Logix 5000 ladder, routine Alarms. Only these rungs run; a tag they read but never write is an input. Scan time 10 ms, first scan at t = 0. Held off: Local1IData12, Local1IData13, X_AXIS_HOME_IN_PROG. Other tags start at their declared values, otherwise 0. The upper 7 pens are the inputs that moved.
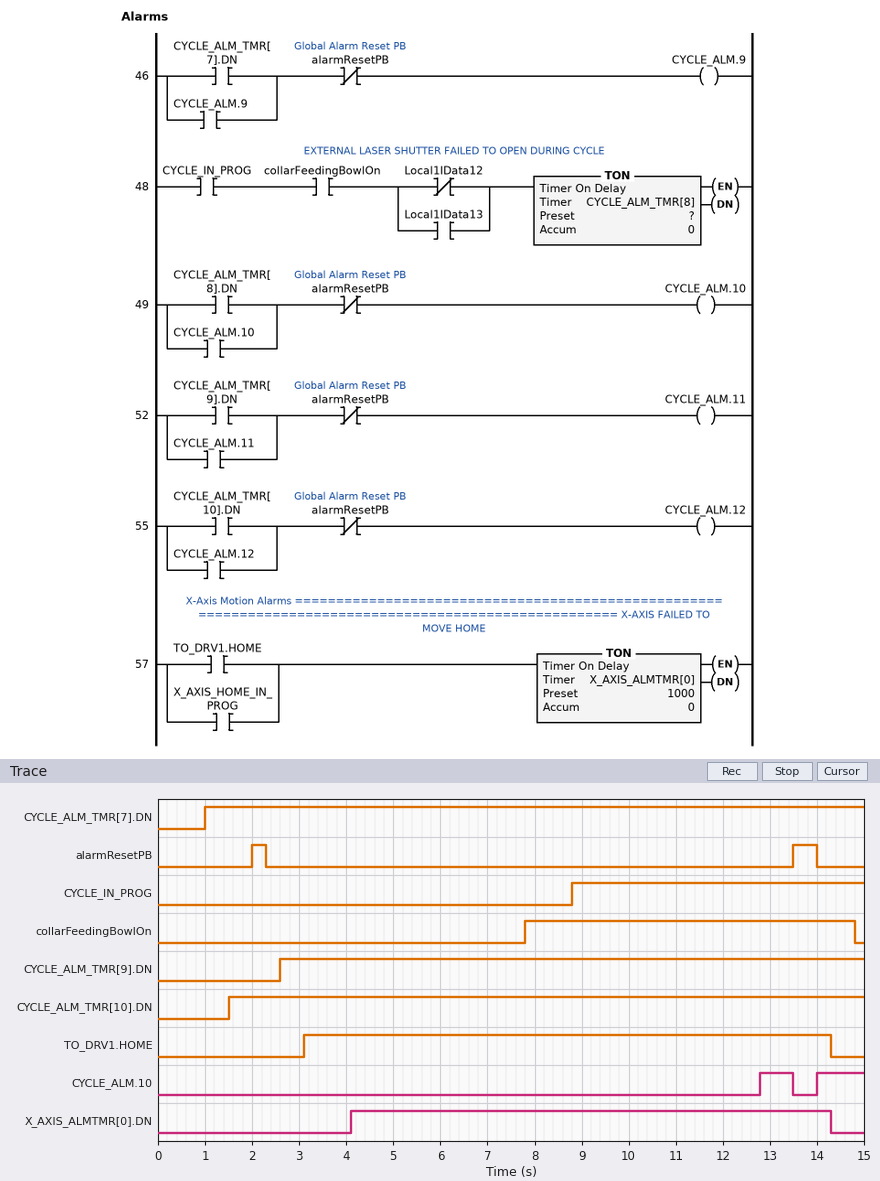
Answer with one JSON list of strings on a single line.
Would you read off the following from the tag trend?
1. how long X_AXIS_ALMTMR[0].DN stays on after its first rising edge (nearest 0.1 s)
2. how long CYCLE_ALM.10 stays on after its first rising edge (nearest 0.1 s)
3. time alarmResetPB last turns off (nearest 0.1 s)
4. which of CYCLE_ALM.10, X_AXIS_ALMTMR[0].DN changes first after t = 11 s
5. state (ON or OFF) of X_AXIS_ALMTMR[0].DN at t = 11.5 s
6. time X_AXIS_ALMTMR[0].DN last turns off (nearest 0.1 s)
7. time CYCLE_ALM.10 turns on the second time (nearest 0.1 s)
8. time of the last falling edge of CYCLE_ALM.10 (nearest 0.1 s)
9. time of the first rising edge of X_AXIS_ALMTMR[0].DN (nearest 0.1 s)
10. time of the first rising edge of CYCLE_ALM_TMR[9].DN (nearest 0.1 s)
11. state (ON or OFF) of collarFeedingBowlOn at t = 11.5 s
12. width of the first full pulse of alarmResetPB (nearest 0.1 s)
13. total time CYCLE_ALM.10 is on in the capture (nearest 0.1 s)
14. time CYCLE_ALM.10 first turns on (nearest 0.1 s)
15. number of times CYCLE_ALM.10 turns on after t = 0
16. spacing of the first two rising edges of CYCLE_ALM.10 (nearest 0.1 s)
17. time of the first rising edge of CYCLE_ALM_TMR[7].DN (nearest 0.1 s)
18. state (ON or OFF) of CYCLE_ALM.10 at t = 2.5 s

["10.2 s", "0.7 s", "14.0 s", "CYCLE_ALM.10", "ON", "14.3 s", "14.0 s", "13.5 s", "4.1 s", "2.6 s", "ON", "0.3 s", "1.7 s", "12.8 s", "2", "1.2 s", "1.0 s", "OFF"]
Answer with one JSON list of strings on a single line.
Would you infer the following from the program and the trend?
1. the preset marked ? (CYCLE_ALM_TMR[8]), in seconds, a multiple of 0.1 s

["4.0 s"]
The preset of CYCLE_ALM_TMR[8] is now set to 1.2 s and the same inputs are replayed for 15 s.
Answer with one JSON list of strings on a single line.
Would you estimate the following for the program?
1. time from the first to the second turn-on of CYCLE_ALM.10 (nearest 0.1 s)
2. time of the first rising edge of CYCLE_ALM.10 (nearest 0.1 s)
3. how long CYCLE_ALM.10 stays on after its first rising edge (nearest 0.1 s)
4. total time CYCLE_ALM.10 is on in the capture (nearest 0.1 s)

["4.0 s", "10.0 s", "3.5 s", "4.5 s"]
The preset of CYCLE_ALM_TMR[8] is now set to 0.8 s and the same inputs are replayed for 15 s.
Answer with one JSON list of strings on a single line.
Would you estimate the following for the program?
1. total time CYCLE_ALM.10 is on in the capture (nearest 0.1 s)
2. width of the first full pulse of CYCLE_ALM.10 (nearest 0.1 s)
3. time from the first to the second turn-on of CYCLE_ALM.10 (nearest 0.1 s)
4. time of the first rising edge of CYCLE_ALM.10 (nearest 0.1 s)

["4.9 s", "3.9 s", "4.4 s", "9.6 s"]
